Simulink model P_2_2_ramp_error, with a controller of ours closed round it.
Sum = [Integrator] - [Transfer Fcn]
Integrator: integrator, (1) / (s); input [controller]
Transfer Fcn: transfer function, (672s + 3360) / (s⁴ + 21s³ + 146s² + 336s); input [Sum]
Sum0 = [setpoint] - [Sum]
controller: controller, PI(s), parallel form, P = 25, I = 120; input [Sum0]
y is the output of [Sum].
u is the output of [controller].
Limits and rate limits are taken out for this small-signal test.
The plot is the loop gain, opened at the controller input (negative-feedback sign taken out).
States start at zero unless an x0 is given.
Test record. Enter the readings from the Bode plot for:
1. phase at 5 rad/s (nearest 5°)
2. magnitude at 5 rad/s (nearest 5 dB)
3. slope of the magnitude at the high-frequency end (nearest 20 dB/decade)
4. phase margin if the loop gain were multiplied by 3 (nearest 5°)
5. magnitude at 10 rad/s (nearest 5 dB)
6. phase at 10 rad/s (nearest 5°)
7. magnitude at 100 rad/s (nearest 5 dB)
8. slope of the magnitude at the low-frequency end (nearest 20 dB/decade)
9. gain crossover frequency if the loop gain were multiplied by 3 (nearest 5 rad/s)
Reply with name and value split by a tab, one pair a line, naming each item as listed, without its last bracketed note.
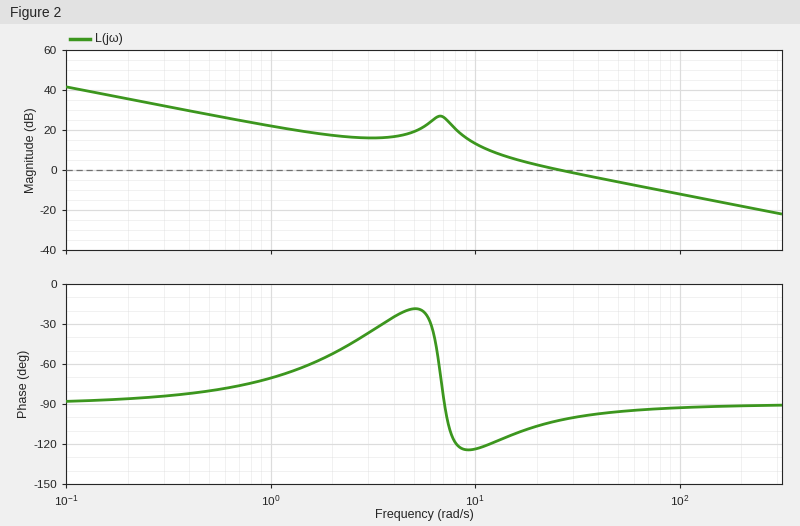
phase at 5 rad/s	-20°
magnitude at 5 rad/s	20 dB
slope of the magnitude at the high-frequency end	-20 dB/decade
phase margin if the loop gain were multiplied by 3	85°
magnitude at 10 rad/s	15 dB
phase at 10 rad/s	-125°
magnitude at 100 rad/s	-10 dB
slope of the magnitude at the low-frequency end	-20 dB/decade
gain crossover frequency if the loop gain were multiplied by 3	75 rad/s
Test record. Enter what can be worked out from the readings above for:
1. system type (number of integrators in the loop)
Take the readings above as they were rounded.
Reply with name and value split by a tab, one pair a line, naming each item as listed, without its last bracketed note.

system type	1
